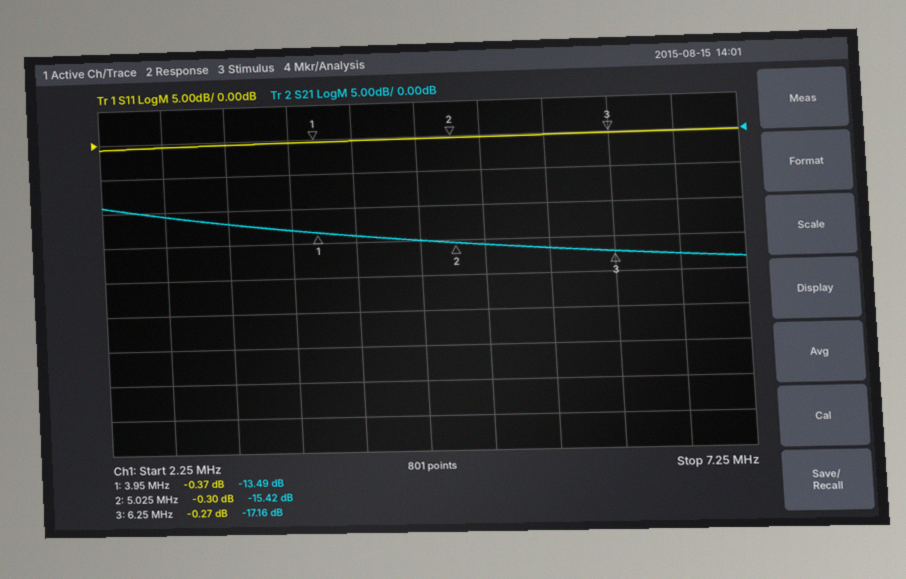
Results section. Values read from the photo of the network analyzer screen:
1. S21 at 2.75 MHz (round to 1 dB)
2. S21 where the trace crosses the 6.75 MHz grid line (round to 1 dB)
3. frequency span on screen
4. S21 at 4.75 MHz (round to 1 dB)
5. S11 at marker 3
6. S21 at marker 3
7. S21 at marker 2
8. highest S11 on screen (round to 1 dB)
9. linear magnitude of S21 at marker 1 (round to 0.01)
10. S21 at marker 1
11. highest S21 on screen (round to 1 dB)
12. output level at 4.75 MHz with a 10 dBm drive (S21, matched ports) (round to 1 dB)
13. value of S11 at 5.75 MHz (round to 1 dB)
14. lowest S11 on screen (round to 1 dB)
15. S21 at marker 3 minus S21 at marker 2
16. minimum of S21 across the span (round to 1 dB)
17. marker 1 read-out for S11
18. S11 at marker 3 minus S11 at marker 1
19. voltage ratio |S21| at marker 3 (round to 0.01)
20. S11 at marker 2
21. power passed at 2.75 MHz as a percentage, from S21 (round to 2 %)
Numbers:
-11 dB
-18 dB
5 MHz
-15 dB
-0.27 dB
-17.16 dB
-15.42 dB
0 dB
0.21
-13.49 dB
-9 dB
-5 dBm
0 dB
-1 dB
-1.74 dB
-18 dB
-0.37 dB
0.10 dB
0.14
-0.30 dB
8 %
